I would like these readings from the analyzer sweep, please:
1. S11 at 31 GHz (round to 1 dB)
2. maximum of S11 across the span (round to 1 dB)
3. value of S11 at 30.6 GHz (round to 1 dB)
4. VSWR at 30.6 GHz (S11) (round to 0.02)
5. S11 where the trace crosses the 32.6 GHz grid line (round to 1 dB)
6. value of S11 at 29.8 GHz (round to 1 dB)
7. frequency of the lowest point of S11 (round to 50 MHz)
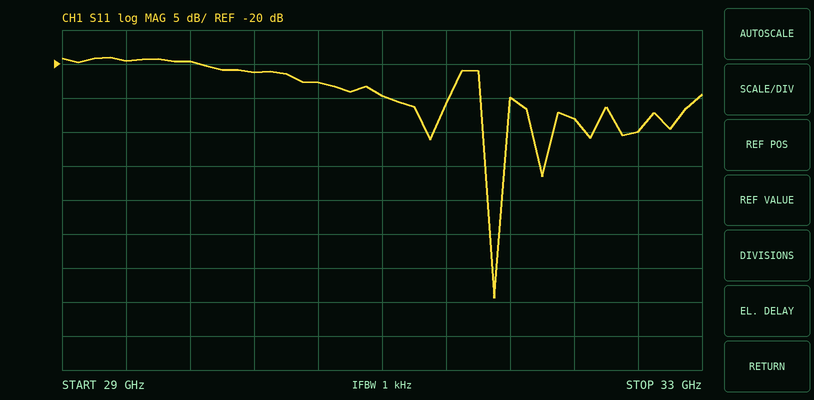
-25 dB
-19 dB
-23 dB
1.16
-30 dB
-20 dB
31.70 GHz
